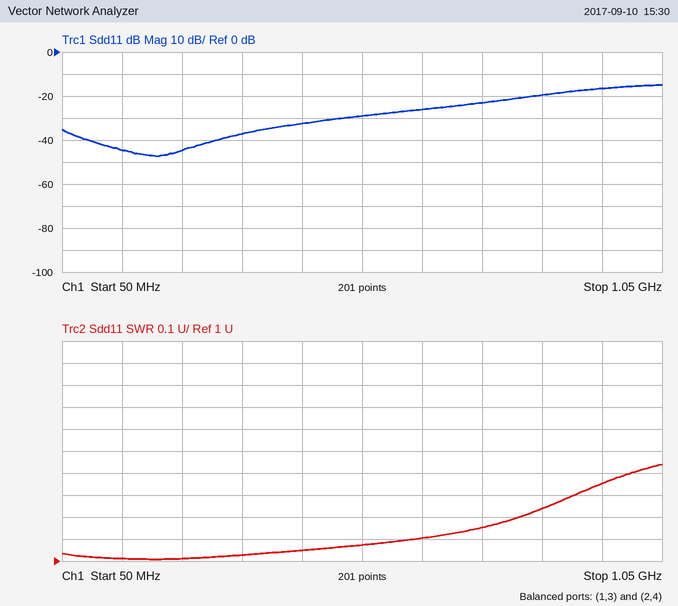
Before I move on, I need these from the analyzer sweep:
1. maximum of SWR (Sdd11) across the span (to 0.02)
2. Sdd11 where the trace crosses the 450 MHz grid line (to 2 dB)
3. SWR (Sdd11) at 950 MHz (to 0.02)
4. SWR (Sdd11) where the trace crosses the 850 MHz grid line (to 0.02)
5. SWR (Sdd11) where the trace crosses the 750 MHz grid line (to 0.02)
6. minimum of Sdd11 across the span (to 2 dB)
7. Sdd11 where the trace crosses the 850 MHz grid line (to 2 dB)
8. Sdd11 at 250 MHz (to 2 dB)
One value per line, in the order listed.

1.44
-32 dB
1.36
1.24
1.16
-48 dB
-20 dB
-44 dB
